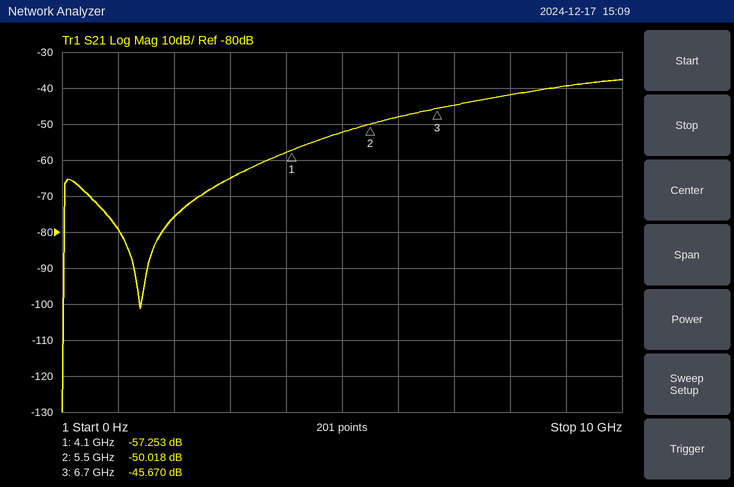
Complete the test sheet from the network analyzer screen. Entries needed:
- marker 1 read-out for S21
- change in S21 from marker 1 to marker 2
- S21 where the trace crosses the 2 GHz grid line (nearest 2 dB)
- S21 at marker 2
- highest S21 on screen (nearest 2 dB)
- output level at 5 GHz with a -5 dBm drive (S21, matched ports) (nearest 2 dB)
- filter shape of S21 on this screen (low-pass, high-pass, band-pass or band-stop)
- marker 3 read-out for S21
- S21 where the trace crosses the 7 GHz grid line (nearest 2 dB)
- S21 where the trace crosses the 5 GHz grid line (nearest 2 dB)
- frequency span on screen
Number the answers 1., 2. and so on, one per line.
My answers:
1. -57.253 dB
2. 7.235 dB
3. -76 dB
4. -50.018 dB
5. -38 dB
6. -58 dBm
7. high-pass
8. -45.670 dB
9. -44 dB
10. -52 dB
11. 10 GHz
